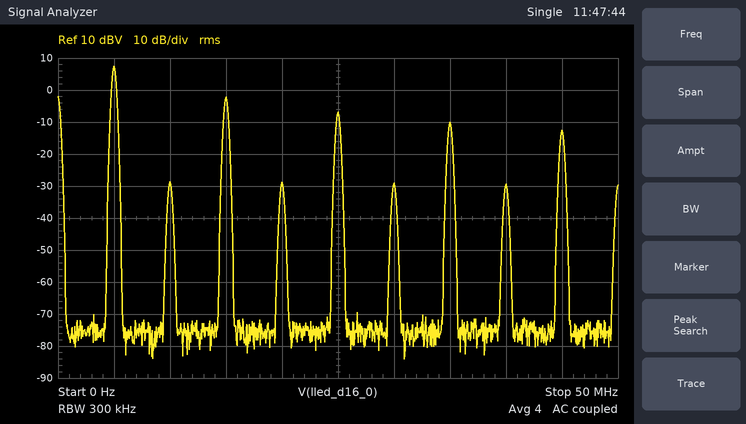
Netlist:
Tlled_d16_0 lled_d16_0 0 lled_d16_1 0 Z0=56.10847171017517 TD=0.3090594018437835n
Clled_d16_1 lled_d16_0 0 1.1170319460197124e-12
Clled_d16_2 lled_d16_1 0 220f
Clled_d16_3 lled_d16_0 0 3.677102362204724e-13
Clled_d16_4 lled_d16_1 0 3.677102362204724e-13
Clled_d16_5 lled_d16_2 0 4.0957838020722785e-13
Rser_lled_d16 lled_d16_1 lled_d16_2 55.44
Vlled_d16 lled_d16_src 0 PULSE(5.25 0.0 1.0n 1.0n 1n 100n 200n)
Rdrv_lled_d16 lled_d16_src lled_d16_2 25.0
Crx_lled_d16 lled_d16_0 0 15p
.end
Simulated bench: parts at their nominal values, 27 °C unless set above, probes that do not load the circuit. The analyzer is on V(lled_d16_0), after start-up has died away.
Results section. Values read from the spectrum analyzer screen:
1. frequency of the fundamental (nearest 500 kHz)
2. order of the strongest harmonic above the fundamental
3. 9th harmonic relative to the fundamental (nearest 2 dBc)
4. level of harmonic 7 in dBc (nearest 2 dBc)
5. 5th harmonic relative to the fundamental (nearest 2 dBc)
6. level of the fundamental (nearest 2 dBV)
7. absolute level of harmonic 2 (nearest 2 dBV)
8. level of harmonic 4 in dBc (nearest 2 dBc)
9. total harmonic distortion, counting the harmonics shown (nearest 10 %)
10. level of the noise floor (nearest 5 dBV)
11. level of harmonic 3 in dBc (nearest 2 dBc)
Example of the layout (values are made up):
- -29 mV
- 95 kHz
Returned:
- 5.0 MHz
- 3
- -20 dBc
- -18 dBc
- -14 dBc
- 8 dBV
- -28 dBV
- -36 dBc
- 40 %
- -75 dBV
- -10 dBc
